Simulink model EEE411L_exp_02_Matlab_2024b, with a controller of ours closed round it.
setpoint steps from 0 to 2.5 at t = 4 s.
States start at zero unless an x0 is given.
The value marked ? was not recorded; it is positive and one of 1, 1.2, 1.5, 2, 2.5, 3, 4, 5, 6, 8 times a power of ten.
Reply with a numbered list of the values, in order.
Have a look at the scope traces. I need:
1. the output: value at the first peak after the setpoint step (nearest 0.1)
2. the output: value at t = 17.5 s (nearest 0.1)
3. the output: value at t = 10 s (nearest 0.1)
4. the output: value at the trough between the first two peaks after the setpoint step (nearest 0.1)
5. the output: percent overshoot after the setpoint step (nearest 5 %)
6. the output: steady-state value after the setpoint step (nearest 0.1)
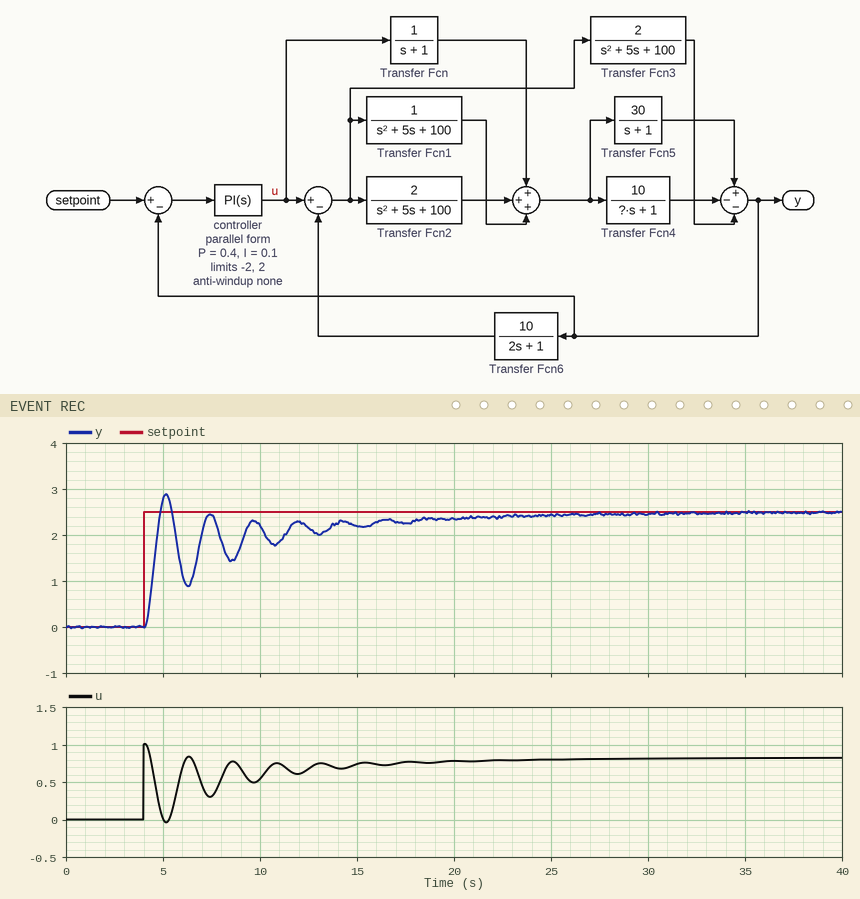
1. 2.9
2. 2.3
3. 2.2
4. 0.9
5. 15 %
6. 2.5
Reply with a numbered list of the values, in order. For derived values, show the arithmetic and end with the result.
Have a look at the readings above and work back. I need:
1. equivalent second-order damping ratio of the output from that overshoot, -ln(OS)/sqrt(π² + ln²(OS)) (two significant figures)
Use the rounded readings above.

1. ln(0.15) = -1.897; 1.897 / sqrt(9.870 + 3.599) = 0.52
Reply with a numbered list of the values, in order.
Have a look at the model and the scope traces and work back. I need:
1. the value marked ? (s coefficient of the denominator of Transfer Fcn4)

1. 0.5
